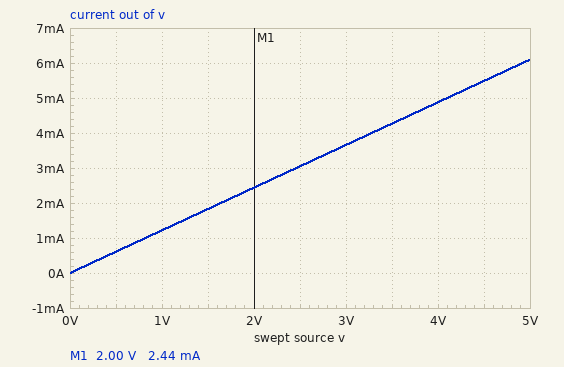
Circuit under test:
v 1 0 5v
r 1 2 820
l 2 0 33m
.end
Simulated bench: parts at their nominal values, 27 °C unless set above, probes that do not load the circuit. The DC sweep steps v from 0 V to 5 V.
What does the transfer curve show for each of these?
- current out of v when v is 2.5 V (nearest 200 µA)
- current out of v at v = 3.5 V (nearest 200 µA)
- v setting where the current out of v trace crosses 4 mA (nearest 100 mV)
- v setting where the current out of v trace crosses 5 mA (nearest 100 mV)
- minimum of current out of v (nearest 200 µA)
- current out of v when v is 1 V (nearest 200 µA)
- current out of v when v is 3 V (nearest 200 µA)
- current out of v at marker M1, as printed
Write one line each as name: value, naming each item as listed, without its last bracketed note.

current out of v when v is 2.5 V: 3.0 mA
current out of v at v = 3.5 V: 4.2 mA
v setting where the current out of v trace crosses 4 mA: 3.3 V
v setting where the current out of v trace crosses 5 mA: 4.1 V
minimum of current out of v: 0 A
current out of v when v is 1 V: 1.2 mA
current out of v when v is 3 V: 3.6 mA
current out of v at marker M1, as printed: 2.44 mA
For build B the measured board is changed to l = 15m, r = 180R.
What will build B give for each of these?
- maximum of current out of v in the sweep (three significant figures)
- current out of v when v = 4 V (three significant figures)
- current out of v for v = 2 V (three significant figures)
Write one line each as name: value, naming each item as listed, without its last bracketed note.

maximum of current out of v in the sweep: 27.8 mA
current out of v when v = 4 V: 22.2 mA
current out of v for v = 2 V: 11.1 mA
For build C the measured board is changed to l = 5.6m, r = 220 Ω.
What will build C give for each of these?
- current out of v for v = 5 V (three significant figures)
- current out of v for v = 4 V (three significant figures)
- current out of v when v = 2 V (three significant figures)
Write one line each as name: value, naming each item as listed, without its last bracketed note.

current out of v for v = 5 V: 22.7 mA
current out of v for v = 4 V: 18.2 mA
current out of v when v = 2 V: 9.09 mA
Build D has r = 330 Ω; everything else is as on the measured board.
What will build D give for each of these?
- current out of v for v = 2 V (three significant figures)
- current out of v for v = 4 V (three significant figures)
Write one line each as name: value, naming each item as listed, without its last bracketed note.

current out of v for v = 2 V: 6.06 mA
current out of v for v = 4 V: 12.1 mA
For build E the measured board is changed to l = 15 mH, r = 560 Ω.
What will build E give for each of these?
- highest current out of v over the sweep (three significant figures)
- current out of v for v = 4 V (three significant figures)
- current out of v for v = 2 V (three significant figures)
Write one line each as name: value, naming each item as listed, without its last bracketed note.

highest current out of v over the sweep: 8.93 mA
current out of v for v = 4 V: 7.14 mA
current out of v for v = 2 V: 3.57 mA
